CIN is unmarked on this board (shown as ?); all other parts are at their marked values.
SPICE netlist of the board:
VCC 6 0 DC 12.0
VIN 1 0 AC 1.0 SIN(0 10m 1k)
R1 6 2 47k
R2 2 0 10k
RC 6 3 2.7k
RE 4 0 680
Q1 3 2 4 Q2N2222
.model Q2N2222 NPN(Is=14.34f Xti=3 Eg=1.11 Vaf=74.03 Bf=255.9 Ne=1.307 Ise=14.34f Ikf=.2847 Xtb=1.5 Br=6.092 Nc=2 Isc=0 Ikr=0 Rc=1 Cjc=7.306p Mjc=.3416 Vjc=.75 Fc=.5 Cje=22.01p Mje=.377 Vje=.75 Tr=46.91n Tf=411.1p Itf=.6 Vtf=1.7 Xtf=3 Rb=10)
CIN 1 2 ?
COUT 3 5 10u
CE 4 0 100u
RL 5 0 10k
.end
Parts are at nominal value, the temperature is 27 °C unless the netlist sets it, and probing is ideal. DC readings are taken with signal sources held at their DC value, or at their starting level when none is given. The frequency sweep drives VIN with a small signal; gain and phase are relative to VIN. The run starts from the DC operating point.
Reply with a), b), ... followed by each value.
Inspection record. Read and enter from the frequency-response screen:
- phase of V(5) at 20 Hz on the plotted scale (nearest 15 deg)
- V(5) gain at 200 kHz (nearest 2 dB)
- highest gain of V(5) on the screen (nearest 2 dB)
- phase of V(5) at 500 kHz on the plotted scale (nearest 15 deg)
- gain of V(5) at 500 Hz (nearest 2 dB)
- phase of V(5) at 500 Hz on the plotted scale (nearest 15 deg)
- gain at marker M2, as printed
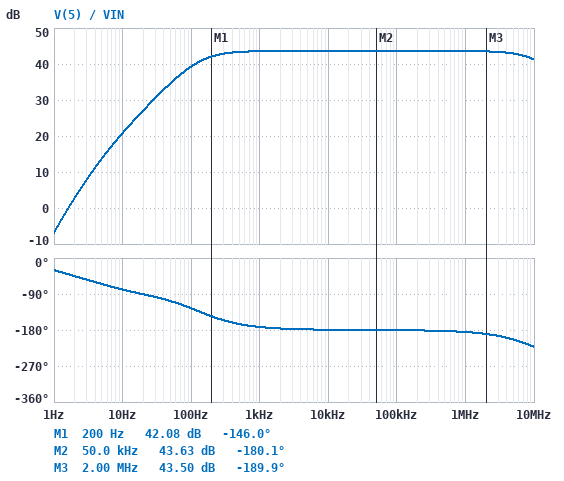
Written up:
a) -90 deg
b) 44 dB
c) 44 dB
d) -180 deg
e) 44 dB
f) -165 deg
g) 43.63 dB
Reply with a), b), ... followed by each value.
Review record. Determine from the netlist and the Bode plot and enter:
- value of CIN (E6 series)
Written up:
a) 4.7 µF
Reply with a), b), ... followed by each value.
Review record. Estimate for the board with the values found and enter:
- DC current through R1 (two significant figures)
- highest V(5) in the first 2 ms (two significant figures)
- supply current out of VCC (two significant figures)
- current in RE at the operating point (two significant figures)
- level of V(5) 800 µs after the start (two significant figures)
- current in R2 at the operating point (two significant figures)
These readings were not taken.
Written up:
a) 210 µA
b) 1.4 V
c) 2.2 mA
d) 2.0 mA
e) 1.3 V
f) 200 µA
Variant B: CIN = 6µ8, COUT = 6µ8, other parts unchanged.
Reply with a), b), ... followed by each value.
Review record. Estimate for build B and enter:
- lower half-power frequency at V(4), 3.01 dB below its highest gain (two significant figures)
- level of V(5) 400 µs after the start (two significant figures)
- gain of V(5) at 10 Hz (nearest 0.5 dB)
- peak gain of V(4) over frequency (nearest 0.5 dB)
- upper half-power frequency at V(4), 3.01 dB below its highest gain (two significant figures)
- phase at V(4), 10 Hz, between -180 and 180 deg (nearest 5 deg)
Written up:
a) 2.7 Hz
b) -580 mV
c) 21.5 dB
d) -1.0 dB
e) 130 Hz
f) 10 deg
